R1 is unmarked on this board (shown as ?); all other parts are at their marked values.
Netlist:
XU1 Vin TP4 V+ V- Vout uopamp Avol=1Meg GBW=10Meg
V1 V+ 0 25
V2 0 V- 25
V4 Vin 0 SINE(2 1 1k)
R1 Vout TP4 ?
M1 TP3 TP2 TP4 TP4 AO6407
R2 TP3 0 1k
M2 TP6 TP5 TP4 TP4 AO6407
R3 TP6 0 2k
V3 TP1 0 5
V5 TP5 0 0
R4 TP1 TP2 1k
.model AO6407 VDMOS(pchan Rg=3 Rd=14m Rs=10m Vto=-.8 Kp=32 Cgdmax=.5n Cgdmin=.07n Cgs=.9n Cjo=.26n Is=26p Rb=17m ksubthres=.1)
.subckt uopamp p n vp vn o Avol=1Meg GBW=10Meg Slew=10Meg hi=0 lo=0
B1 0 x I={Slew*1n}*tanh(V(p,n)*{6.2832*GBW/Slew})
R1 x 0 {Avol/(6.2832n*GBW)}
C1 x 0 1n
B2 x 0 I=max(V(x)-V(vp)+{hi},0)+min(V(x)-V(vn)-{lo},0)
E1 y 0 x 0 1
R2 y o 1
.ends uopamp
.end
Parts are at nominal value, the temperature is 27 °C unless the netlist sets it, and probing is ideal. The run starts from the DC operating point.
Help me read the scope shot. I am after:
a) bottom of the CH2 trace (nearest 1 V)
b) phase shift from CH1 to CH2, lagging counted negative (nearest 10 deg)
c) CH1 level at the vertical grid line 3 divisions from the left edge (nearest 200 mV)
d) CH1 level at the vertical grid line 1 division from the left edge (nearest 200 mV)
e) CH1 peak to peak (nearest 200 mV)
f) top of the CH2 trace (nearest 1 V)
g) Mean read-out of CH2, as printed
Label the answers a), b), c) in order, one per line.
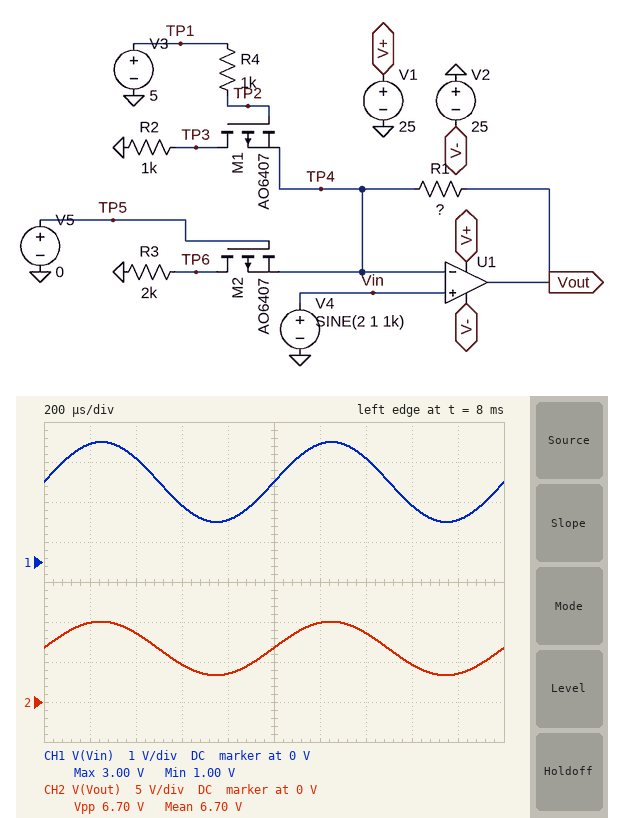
a) 3 V
b) 0 deg
c) 1.4 V
d) 3.0 V
e) 2.0 V
f) 10 V
g) 6.70 V
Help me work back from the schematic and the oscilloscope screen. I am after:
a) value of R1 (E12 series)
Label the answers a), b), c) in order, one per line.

a) 4.7 kΩ
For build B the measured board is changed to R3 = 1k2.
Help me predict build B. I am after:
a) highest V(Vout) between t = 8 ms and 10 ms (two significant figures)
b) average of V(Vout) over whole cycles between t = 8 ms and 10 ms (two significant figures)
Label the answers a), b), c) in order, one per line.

a) 15 V
b) 9.8 V
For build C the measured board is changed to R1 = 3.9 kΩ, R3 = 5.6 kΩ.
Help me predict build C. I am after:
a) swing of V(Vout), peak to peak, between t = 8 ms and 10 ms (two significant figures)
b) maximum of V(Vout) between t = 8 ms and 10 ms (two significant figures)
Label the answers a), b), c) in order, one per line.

a) 3.4 V
b) 5.1 V
